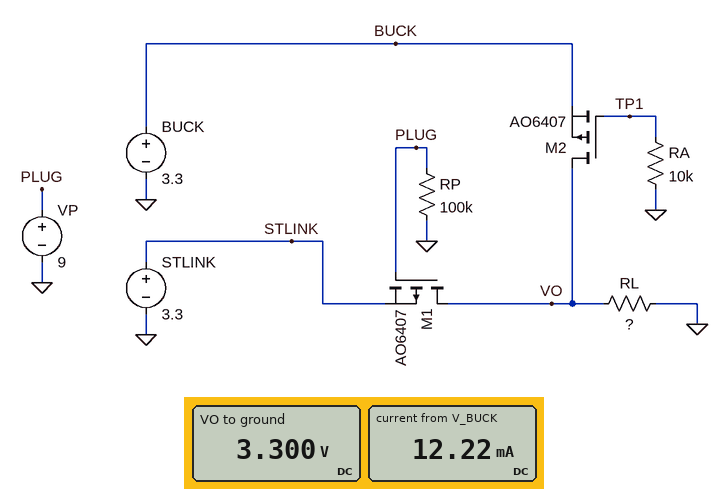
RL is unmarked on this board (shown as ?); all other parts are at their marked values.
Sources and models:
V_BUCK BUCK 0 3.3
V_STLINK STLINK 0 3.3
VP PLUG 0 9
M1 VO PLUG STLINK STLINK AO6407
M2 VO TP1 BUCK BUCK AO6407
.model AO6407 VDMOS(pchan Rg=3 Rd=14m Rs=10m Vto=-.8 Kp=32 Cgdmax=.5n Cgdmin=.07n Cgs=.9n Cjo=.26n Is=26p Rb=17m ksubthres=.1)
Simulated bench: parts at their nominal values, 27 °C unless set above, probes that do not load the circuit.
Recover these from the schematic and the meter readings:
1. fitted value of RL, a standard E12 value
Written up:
270 Ω
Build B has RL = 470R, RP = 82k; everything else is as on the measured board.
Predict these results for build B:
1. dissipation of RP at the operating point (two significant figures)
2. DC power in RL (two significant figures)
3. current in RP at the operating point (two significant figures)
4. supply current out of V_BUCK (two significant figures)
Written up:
990 µW
23 mW
110 µA
7.0 mA
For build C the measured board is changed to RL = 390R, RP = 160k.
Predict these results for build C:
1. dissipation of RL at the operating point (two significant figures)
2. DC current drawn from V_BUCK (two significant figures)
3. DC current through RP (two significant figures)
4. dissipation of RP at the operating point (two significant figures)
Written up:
28 mW
8.5 mA
56 µA
510 µW
